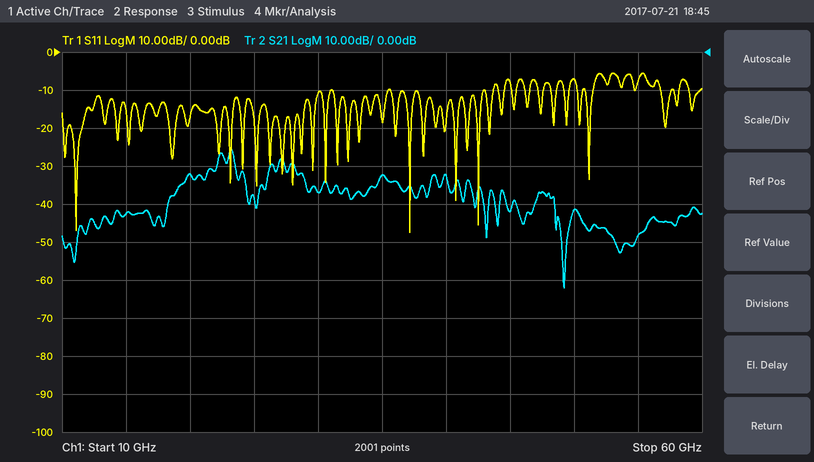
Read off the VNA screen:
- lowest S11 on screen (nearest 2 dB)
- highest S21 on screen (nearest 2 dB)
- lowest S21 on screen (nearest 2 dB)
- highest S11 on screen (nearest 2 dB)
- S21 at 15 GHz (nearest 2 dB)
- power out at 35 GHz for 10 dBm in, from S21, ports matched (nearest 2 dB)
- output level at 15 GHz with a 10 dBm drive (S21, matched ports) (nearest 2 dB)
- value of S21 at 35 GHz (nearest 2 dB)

-48 dB
-26 dB
-62 dB
-6 dB
-42 dB
-22 dBm
-32 dBm
-32 dB
